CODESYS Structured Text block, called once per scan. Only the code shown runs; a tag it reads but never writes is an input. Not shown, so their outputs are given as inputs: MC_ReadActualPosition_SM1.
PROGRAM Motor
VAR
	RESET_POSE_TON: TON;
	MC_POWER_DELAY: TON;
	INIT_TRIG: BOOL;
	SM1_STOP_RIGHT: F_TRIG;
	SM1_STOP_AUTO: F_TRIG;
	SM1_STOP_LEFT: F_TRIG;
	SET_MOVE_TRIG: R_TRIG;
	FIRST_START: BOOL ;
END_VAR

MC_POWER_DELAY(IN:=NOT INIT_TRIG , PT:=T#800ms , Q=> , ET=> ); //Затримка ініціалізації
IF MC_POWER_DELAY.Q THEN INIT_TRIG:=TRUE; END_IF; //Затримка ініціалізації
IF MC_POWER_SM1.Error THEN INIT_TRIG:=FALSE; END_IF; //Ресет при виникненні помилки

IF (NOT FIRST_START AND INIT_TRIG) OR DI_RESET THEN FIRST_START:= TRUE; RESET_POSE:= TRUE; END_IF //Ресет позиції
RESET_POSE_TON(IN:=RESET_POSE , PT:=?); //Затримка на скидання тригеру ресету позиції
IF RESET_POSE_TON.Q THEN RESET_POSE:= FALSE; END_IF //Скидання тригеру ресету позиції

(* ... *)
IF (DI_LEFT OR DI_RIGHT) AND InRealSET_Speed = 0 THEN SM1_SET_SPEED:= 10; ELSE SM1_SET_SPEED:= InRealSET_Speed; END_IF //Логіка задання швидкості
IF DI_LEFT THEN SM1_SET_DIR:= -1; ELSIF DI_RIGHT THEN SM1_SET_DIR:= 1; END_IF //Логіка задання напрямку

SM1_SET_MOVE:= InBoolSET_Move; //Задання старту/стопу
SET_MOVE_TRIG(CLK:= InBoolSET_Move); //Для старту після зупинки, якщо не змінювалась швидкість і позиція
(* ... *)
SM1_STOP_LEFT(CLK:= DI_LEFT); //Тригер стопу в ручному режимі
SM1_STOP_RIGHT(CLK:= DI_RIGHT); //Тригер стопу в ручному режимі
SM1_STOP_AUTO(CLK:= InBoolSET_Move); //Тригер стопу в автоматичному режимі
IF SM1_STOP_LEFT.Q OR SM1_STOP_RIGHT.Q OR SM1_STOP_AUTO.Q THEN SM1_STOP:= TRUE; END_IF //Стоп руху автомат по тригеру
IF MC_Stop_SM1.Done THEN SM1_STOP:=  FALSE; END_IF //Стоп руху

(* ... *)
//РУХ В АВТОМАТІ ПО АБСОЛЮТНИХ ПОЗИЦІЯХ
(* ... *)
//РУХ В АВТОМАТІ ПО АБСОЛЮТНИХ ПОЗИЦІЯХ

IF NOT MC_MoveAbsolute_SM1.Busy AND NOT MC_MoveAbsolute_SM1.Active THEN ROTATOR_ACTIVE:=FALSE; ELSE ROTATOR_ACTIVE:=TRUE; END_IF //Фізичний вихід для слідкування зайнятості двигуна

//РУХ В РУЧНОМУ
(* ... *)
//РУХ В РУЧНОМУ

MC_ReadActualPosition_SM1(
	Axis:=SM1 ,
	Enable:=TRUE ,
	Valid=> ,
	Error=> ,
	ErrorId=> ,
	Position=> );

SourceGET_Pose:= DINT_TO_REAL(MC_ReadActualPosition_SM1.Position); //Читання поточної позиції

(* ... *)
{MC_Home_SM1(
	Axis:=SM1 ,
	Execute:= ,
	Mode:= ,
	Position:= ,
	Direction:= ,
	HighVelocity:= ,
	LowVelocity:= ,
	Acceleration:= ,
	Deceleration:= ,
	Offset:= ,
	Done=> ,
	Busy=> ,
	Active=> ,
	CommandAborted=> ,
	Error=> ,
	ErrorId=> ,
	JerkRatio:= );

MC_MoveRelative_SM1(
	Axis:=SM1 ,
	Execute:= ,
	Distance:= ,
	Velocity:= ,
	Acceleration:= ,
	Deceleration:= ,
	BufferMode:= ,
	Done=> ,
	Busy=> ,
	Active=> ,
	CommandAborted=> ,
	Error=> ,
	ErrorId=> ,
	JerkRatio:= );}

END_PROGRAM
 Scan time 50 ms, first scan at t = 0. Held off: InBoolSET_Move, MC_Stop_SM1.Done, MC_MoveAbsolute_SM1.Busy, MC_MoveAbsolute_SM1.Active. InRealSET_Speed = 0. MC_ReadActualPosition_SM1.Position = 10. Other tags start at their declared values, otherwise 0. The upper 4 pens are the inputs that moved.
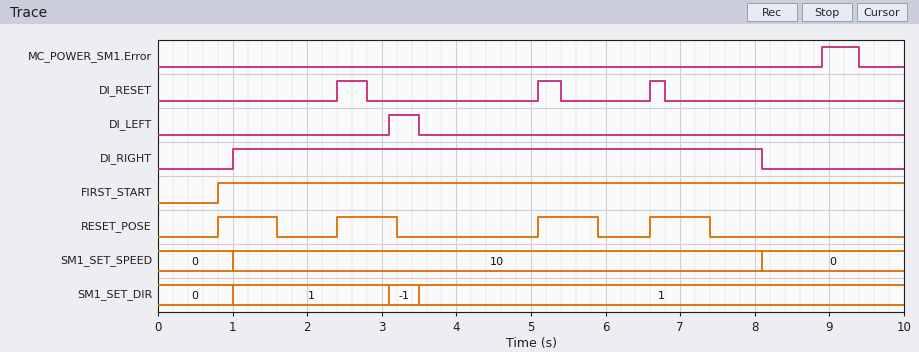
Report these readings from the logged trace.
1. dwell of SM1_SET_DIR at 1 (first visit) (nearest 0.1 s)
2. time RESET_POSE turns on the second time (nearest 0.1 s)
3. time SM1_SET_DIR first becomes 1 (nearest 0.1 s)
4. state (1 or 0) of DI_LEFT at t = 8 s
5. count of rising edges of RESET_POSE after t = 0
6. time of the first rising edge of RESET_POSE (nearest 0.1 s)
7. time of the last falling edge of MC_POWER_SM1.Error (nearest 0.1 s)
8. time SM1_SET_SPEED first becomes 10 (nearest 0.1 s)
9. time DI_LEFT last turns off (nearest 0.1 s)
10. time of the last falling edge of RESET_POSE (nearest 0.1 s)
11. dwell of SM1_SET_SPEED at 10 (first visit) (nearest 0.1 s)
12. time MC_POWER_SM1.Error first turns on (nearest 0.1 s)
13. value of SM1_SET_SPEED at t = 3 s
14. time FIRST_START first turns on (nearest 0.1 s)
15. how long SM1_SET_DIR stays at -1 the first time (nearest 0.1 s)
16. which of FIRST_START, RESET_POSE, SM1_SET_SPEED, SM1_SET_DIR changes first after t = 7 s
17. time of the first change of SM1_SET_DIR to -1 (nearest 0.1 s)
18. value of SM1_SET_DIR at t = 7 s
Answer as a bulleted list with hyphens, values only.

- 2.1 s
- 2.4 s
- 1.0 s
- 0
- 4
- 0.8 s
- 9.4 s
- 1.0 s
- 3.5 s
- 7.4 s
- 7.1 s
- 8.9 s
- 10
- 0.8 s
- 0.4 s
- RESET_POSE
- 3.1 s
- 1
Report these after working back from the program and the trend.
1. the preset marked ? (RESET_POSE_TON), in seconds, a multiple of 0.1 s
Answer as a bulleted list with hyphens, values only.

- 0.8 s
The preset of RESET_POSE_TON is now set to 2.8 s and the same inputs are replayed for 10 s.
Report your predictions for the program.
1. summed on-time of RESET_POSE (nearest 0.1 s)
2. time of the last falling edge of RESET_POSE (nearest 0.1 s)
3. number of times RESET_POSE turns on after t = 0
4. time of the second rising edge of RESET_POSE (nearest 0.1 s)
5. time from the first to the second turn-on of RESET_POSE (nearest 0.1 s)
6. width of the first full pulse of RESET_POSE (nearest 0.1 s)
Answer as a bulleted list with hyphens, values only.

- 5.6 s
- 7.9 s
- 2
- 5.1 s
- 4.3 s
- 2.8 s
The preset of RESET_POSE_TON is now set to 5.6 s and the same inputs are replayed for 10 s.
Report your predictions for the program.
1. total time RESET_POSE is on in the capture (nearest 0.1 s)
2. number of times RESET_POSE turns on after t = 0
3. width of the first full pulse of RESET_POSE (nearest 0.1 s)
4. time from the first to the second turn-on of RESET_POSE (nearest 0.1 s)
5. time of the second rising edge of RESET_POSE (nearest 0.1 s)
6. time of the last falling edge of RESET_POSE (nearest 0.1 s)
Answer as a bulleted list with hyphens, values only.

- 9.0 s
- 2
- 5.6 s
- 5.8 s
- 6.6 s
- 6.4 s
